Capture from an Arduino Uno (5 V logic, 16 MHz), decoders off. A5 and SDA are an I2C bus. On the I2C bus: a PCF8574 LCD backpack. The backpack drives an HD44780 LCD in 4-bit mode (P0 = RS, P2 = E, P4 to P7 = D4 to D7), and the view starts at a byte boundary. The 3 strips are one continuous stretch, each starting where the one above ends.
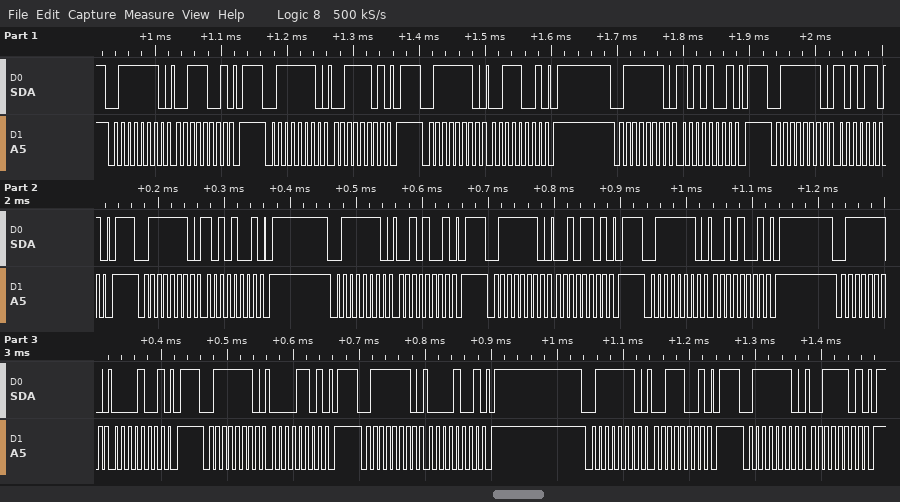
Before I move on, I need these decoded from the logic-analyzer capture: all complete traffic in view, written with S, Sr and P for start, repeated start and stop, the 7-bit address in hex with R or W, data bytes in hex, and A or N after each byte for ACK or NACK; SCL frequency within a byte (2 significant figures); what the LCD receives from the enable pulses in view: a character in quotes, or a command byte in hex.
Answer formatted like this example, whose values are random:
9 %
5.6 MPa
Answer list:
S 3FW A 39 A P S 3FW A 3D A P S 3FW A 39 A P S 3FW A A9 A P S 3FW A AD A P S 3FW A A9 A P S 3FW A 29 A P S 3FW A 2D A P S 3FW A 29 A P S 3FW A 09 A P S 3FW A 0D A P S 3FW A 09 A P S 3FW A 39 A P S 3FW A 3D A P
100 kHz
':' ' '
